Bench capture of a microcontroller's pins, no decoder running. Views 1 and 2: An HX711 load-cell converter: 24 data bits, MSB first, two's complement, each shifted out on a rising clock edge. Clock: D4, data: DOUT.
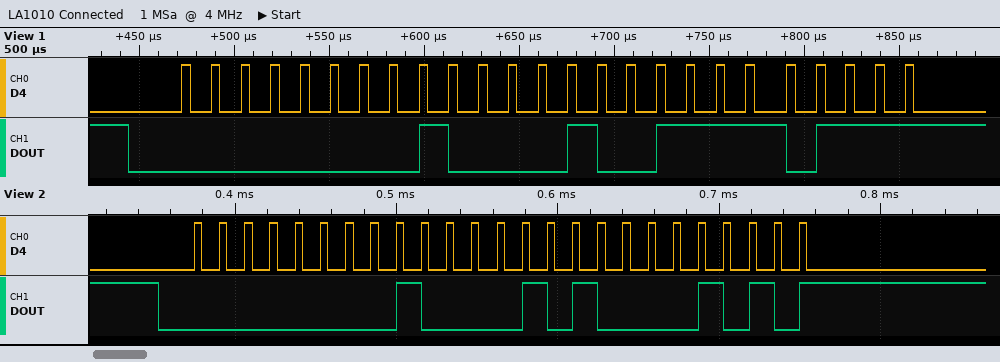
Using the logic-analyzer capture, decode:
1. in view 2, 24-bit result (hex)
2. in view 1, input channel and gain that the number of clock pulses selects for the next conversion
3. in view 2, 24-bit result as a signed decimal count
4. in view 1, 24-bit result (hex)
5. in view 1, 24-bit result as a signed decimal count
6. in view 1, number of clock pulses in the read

0x00850A
channel A, gain 128
34058
0x0084F7
34039
25
